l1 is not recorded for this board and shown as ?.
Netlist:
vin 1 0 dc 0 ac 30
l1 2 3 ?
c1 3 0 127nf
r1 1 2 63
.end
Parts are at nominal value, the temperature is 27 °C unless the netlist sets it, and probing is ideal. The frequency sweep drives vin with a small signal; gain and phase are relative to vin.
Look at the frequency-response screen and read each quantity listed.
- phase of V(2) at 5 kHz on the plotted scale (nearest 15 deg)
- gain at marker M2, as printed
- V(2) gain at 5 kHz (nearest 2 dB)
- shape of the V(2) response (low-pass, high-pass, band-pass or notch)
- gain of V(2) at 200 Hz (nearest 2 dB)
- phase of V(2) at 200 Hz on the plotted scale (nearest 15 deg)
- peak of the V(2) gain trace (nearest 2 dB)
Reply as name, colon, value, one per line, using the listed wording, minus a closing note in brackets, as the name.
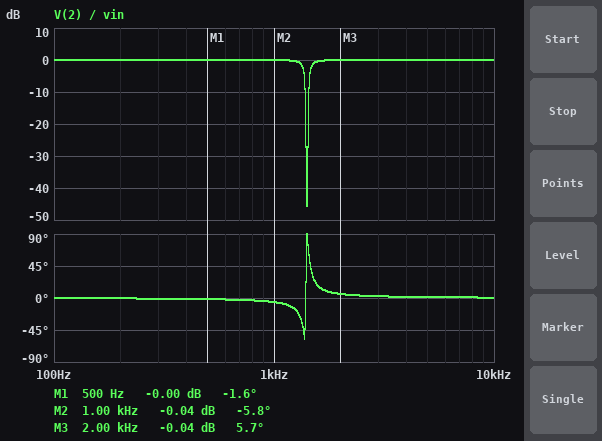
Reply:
phase of V(2) at 5 kHz on the plotted scale: 0 deg
gain at marker M2, as printed: -0.04 dB
V(2) gain at 5 kHz: 0 dB
shape of the V(2) response: notch
gain of V(2) at 200 Hz: 0 dB
phase of V(2) at 200 Hz on the plotted scale: 0 deg
peak of the V(2) gain trace: 0 dB
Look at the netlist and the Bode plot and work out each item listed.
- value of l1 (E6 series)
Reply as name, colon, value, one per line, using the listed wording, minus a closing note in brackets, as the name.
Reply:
value of l1: 100 mH
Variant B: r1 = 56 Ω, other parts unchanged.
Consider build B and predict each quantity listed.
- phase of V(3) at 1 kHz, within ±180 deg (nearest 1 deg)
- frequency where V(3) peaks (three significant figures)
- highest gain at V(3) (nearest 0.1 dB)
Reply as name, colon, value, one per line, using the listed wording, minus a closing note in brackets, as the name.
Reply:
phase of V(3) at 1 kHz, within ±180 deg: -5 deg
frequency where V(3) peaks: 1.41 kHz
highest gain at V(3): 24.0 dB
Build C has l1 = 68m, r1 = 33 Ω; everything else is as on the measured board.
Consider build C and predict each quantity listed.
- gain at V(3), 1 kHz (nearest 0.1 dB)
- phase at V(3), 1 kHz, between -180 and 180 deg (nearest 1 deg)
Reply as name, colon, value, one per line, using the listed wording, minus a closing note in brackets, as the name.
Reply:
gain at V(3), 1 kHz: 3.6 dB
phase at V(3), 1 kHz, between -180 and 180 deg: -2 deg
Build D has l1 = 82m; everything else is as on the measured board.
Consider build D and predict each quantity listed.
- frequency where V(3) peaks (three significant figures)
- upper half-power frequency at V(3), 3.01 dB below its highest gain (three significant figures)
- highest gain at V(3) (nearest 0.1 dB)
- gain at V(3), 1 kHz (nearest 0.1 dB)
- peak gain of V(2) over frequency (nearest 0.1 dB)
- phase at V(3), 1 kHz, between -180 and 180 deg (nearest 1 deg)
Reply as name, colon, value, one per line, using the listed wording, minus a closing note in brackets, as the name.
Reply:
frequency where V(3) peaks: 1.56 kHz
upper half-power frequency at V(3), 3.01 dB below its highest gain: 1.62 kHz
highest gain at V(3): 22.1 dB
gain at V(3), 1 kHz: 4.6 dB
peak gain of V(2) over frequency: 0 dB
phase at V(3), 1 kHz, between -180 and 180 deg: -5 deg
